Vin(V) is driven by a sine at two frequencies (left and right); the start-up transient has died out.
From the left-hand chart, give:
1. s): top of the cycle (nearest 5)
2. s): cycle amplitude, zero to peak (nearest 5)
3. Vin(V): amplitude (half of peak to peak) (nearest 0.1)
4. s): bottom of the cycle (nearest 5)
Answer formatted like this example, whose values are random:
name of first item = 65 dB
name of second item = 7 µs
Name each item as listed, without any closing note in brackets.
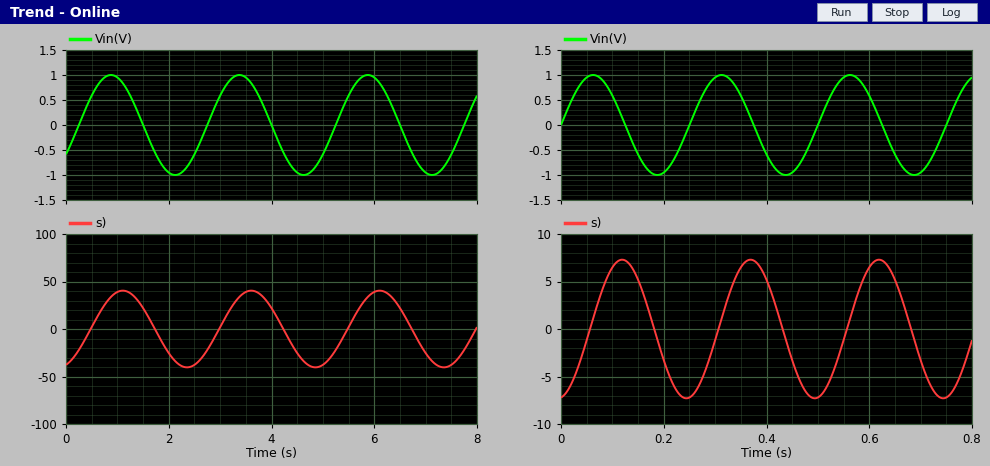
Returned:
s): top of the cycle = 40
s): cycle amplitude, zero to peak = 40
Vin(V): amplitude (half of peak to peak) = 1.0
s): bottom of the cycle = -40
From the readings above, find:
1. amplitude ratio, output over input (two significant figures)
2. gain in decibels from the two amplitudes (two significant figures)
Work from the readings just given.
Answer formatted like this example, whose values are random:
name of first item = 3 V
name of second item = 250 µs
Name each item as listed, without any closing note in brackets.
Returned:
amplitude ratio, output over input = 40
gain in decibels from the two amplitudes = 32 dB
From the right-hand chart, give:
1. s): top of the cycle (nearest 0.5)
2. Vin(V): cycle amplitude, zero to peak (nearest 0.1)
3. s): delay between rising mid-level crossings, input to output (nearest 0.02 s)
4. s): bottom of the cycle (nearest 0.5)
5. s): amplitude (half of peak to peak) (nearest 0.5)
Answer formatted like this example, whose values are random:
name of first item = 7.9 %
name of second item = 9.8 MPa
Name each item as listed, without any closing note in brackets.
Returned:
s): top of the cycle = 7.5
Vin(V): cycle amplitude, zero to peak = 1.0
s): delay between rising mid-level crossings, input to output = 0.06 s
s): bottom of the cycle = -7.5
s): amplitude (half of peak to peak) = 7.5
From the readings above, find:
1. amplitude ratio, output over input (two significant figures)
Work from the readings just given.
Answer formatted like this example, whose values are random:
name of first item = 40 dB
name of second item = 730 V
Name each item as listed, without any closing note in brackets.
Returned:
amplitude ratio, output over input = 7.5
